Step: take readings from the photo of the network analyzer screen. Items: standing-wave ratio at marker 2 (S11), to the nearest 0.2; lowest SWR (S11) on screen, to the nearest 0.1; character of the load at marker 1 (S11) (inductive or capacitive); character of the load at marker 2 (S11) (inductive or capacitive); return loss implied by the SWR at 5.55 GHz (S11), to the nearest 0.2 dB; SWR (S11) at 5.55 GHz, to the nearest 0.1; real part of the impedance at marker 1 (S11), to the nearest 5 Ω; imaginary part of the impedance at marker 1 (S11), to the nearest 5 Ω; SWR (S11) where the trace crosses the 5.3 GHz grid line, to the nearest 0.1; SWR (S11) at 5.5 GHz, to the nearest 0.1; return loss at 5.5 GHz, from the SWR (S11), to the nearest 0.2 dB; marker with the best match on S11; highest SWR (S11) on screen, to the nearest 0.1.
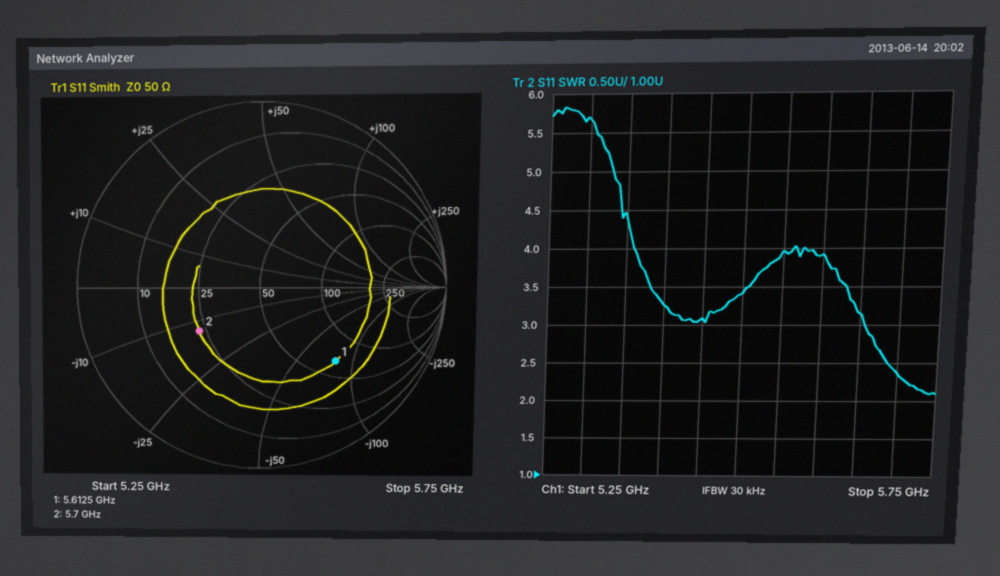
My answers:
2.4
2.1
capacitive
capacitive
4.4 dB
4.0
65 Ω
-80 Ω
5.7
3.4
5.2 dB
marker 2
5.8
